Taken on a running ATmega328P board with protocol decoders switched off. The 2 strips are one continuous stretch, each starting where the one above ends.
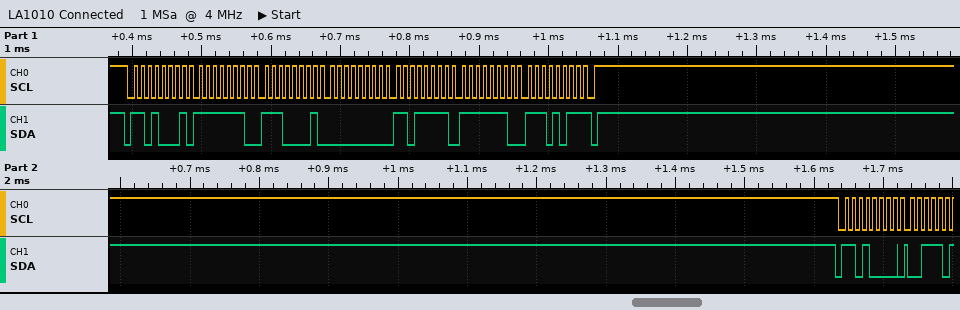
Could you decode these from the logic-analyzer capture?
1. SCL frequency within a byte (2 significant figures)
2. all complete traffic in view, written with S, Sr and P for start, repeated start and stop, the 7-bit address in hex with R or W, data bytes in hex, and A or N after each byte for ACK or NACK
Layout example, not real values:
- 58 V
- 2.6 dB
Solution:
- 100 kHz
- S 68R A FE A E1 A 00 A DF A FE A EB N P S 68W A
